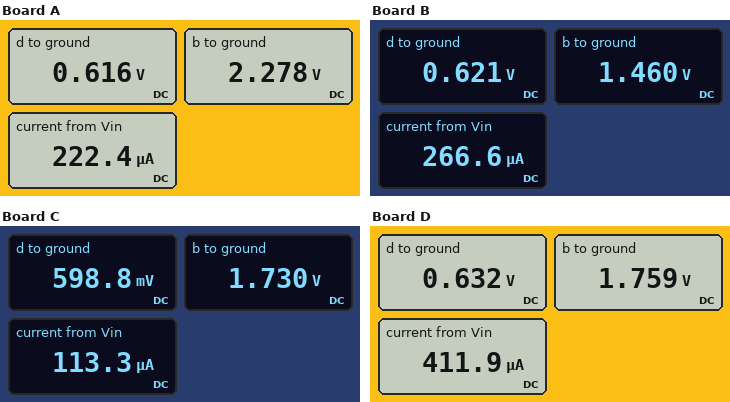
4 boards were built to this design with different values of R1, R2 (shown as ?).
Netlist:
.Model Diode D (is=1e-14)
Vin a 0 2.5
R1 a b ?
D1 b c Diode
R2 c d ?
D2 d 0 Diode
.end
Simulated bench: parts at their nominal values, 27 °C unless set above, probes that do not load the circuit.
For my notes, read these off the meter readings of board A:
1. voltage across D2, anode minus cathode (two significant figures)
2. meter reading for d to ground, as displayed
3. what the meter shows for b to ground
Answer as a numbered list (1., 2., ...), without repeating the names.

1. 620 mV
2. 0.616 V
3. 2.278 V
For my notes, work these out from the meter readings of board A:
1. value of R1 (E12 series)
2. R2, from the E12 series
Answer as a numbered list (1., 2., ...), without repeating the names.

1. 1 kΩ
2. 4.7 kΩ
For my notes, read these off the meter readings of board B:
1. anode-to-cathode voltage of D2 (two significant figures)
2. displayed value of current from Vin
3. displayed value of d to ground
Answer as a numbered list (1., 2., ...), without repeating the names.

1. 620 mV
2. 266.6 µA
3. 0.621 V
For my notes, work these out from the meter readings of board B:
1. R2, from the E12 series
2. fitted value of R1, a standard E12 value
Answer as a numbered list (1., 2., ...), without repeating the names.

1. 820 Ω
2. 3.9 kΩ
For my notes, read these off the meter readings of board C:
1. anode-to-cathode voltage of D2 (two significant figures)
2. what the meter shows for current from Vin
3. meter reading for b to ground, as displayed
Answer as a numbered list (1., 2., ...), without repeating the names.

1. 600 mV
2. 113.3 µA
3. 1.730 V
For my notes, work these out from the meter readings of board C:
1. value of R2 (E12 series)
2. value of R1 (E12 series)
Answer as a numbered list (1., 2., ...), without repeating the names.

1. 4.7 kΩ
2. 6.8 kΩ
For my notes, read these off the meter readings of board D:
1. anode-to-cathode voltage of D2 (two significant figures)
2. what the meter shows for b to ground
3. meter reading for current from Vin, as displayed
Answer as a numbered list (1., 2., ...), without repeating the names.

1. 630 mV
2. 1.759 V
3. 411.9 µA
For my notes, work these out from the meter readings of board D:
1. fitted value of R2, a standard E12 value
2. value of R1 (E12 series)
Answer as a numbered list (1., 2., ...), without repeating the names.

1. 1.2 kΩ
2. 1.8 kΩ
